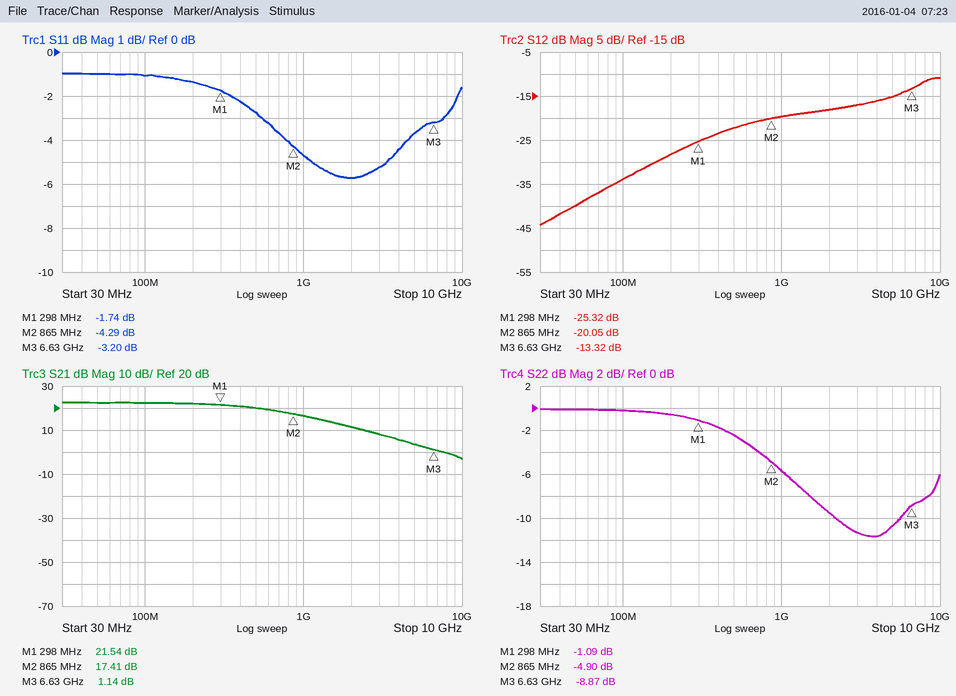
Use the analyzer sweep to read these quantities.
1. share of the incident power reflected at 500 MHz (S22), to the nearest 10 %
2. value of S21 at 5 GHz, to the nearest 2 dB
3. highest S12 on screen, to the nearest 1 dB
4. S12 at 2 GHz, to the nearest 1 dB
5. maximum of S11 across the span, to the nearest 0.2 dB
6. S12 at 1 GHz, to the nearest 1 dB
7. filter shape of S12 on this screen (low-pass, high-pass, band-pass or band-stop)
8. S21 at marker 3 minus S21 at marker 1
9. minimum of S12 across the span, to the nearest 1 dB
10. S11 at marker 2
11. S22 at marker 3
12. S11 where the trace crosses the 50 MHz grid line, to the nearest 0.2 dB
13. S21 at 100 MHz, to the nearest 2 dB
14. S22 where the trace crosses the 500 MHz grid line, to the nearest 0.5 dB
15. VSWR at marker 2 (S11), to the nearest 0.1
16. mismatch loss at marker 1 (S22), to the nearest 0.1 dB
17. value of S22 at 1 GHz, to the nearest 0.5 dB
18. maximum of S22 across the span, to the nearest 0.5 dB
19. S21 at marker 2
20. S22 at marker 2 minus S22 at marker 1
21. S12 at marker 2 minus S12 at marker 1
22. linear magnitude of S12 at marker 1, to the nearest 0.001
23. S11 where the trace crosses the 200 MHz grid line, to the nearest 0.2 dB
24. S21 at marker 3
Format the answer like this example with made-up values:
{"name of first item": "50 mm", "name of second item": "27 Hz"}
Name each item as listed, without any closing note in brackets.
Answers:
{"share of the incident power reflected at 500 MHz (S22), to the nearest 10 %": "60 %", "value of S21 at 5 GHz, to the nearest 2 dB": "4 dB", "highest S12 on screen, to the nearest 1 dB": "-11 dB", "S12 at 2 GHz, to the nearest 1 dB": "-18 dB", "maximum of S11 across the span, to the nearest 0.2 dB": "-1.0 dB", "S12 at 1 GHz, to the nearest 1 dB": "-20 dB", "filter shape of S12 on this screen": "high-pass", "S21 at marker 3 minus S21 at marker 1": "-20.40 dB", "minimum of S12 across the span, to the nearest 1 dB": "-44 dB", "S11 at marker 2": "-4.29 dB", "S22 at marker 3": "-8.87 dB", "S11 where the trace crosses the 50 MHz grid line, to the nearest 0.2 dB": "-1.0 dB", "S21 at 100 MHz, to the nearest 2 dB": "22 dB", "S22 where the trace crosses the 500 MHz grid line, to the nearest 0.5 dB": "-2.5 dB", "VSWR at marker 2 (S11), to the nearest 0.1": "4.1", "mismatch loss at marker 1 (S22), to the nearest 0.1 dB": "6.5 dB", "value of S22 at 1 GHz, to the nearest 0.5 dB": "-5.5 dB", "maximum of S22 across the span, to the nearest 0.5 dB": "0.0 dB", "S21 at marker 2": "17.41 dB", "S22 at marker 2 minus S22 at marker 1": "-3.81 dB", "S12 at marker 2 minus S12 at marker 1": "5.27 dB", "linear magnitude of S12 at marker 1, to the nearest 0.001": "0.054", "S11 where the trace crosses the 200 MHz grid line, to the nearest 0.2 dB": "-1.4 dB", "S21 at marker 3": "1.14 dB"}
